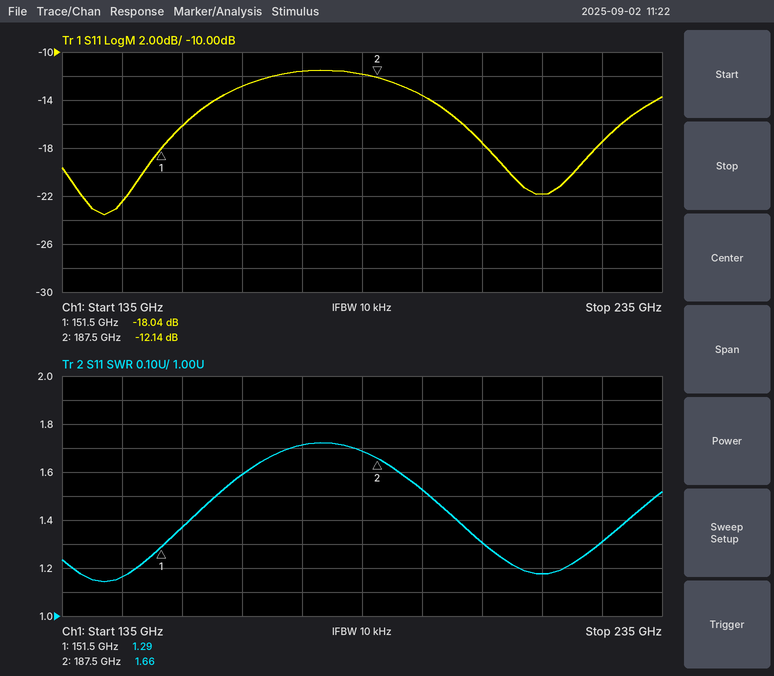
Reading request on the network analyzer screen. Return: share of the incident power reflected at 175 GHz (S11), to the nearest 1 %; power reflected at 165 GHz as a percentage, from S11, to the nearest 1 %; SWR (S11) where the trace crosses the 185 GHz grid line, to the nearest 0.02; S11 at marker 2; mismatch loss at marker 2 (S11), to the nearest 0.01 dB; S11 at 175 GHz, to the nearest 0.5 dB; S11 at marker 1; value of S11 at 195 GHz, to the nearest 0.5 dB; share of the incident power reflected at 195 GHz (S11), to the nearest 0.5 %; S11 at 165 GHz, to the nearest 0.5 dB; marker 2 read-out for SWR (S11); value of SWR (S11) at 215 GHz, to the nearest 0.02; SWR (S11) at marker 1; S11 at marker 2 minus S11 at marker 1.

7 %
5 %
1.68
-12.14 dB
0.27 dB
-11.5 dB
-18.04 dB
-13.5 dB
4.5 %
-13.0 dB
1.66
1.18
1.29
5.90 dB
